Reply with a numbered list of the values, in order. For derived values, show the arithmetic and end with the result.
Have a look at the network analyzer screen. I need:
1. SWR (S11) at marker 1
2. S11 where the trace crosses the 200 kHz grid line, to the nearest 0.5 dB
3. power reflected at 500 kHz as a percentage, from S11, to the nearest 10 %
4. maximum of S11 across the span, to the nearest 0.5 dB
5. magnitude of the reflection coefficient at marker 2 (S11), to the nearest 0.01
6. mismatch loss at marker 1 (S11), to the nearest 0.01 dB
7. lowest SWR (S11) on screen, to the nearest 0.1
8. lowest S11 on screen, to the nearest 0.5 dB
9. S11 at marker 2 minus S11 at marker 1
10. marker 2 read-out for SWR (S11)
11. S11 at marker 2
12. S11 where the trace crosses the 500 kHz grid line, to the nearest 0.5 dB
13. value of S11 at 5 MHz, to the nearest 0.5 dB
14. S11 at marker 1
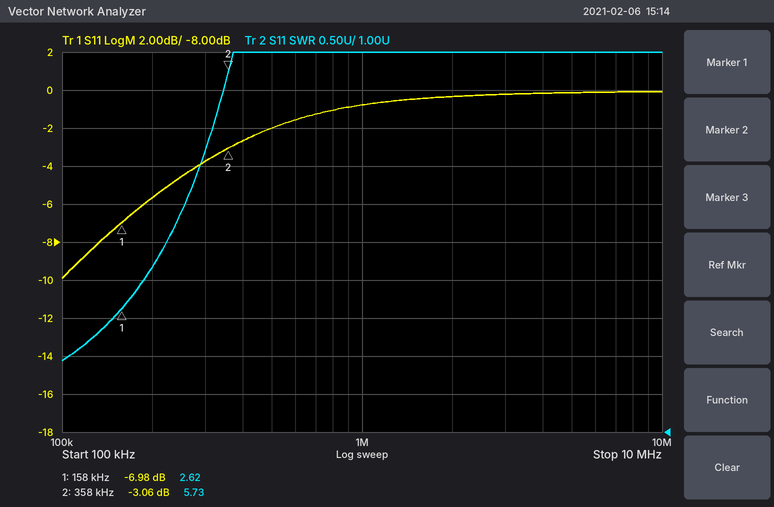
1. 2.62
2. -5.5 dB
3. 10^(-2/10) ≈ 63.1 %, so 60 % to the nearest 10 %
4. 0.0 dB
5. 10^(-3.06/20) ≈ 0.70
6. −10 log10(1 − 10^(-6.98/10)) ≈ 0.97 dB
7. 1.9
8. -10.0 dB
9. -3.06 − (-6.98) = 3.92 dB
10. 5.73
11. -3.06 dB
12. -2.0 dB
13. 0.0 dB
14. -6.98 dB
